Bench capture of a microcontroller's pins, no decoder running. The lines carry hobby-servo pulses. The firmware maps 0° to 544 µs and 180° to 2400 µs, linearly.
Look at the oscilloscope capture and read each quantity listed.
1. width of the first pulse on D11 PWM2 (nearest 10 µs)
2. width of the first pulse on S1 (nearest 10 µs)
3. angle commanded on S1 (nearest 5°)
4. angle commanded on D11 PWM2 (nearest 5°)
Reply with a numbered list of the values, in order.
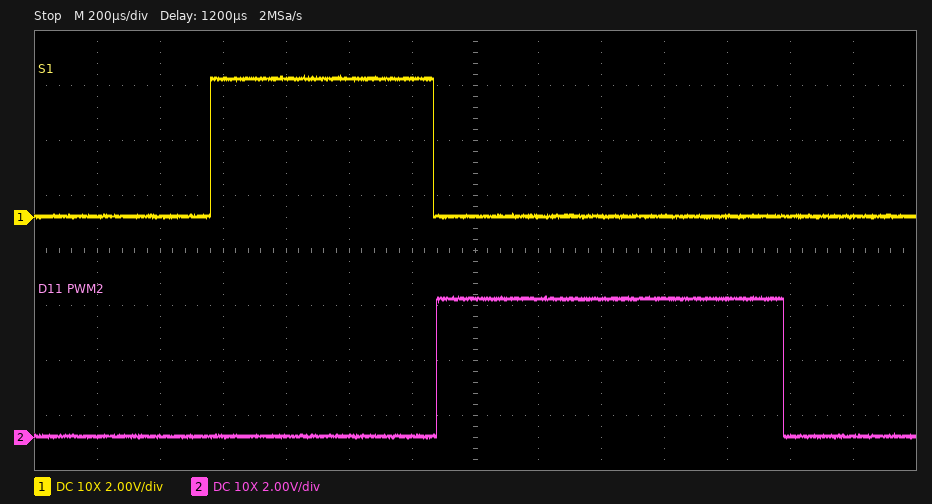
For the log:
1. 1100 µs
2. 710 µs
3. 15°
4. 55°
